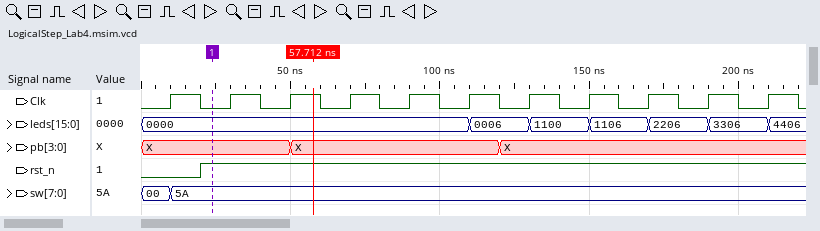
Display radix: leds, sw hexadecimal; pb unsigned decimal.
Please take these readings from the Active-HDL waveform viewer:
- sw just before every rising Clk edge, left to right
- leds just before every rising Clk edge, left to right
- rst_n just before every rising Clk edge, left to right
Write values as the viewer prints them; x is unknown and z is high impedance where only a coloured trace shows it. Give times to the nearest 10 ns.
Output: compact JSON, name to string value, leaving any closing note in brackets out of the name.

{"sw just before every rising Clk edge, left to right": "00, 5A, 5A, 5A, 5A, 5A, 5A, 5A, 5A, 5A, 5A", "leds just before every rising Clk edge, left to right": "0000, 0000, 0000, 0000, 0000, 0000, 0006, 1100, 1106, 2206, 3306", "rst_n just before every rising Clk edge, left to right": "0 1 1 1 1 1 1 1 1 1 1"}
